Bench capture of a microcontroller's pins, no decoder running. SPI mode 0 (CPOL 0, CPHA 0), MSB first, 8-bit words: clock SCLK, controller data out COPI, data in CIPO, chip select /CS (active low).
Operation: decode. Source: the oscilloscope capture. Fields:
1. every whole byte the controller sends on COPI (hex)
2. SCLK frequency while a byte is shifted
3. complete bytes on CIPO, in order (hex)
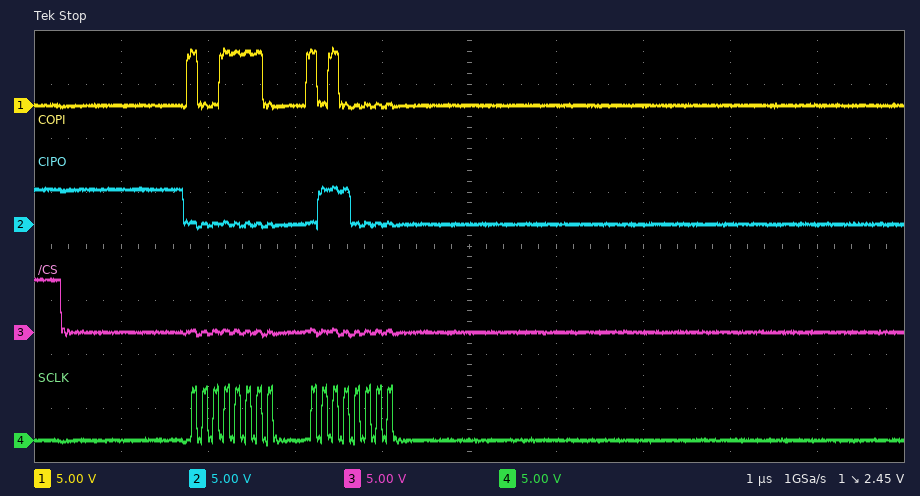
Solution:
9E A0
8 MHz
00 70
